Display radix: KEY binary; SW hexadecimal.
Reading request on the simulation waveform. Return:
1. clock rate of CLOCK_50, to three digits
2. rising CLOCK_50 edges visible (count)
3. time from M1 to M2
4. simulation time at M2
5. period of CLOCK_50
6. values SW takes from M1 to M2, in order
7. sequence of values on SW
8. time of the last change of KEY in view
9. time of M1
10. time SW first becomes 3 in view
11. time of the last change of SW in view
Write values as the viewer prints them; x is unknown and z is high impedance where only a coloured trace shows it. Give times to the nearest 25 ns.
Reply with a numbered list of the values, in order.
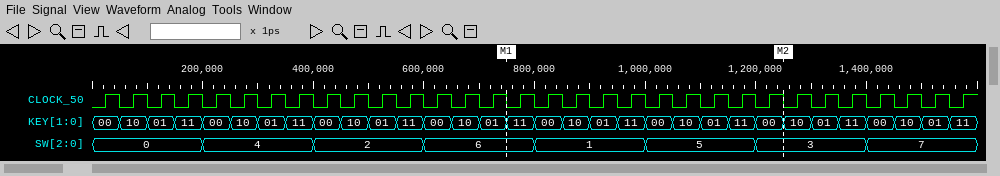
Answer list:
1. 20.0 MHz
2. 32
3. 500 ns
4. 1250 ns
5. 50 ns
6. 6, 1, 5, 3
7. 0, 4, 2, 6, 1, 5, 3, 7
8. 1550 ns
9. 750 ns
10. 1200 ns
11. 1400 ns
